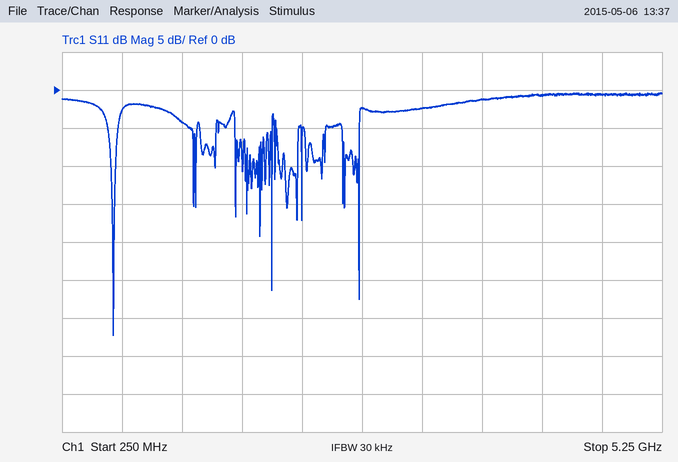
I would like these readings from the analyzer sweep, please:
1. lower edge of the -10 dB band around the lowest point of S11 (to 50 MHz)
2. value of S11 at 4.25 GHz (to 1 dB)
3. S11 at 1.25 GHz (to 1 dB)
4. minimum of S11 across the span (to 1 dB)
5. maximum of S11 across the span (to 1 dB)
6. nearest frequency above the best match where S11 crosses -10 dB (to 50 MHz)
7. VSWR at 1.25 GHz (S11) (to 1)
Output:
650 MHz
-1 dB
-4 dB
-32 dB
0 dB
700 MHz
4
